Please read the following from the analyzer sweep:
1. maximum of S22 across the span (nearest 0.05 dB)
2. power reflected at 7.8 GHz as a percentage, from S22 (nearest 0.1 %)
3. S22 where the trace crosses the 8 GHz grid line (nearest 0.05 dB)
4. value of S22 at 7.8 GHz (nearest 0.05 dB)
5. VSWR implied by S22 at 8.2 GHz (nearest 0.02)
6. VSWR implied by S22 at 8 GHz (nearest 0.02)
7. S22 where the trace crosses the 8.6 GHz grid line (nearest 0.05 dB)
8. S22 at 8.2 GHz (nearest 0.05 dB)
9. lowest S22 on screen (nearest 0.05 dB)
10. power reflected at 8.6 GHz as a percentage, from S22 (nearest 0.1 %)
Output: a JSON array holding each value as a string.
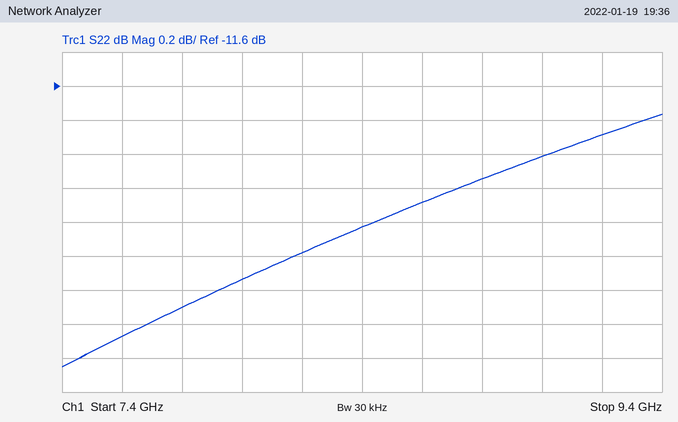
["-11.75 dB", "5.1 %", "-12.75 dB", "-12.90 dB", "1.62", "1.60", "-12.30 dB", "-12.60 dB", "-13.25 dB", "5.9 %"]
